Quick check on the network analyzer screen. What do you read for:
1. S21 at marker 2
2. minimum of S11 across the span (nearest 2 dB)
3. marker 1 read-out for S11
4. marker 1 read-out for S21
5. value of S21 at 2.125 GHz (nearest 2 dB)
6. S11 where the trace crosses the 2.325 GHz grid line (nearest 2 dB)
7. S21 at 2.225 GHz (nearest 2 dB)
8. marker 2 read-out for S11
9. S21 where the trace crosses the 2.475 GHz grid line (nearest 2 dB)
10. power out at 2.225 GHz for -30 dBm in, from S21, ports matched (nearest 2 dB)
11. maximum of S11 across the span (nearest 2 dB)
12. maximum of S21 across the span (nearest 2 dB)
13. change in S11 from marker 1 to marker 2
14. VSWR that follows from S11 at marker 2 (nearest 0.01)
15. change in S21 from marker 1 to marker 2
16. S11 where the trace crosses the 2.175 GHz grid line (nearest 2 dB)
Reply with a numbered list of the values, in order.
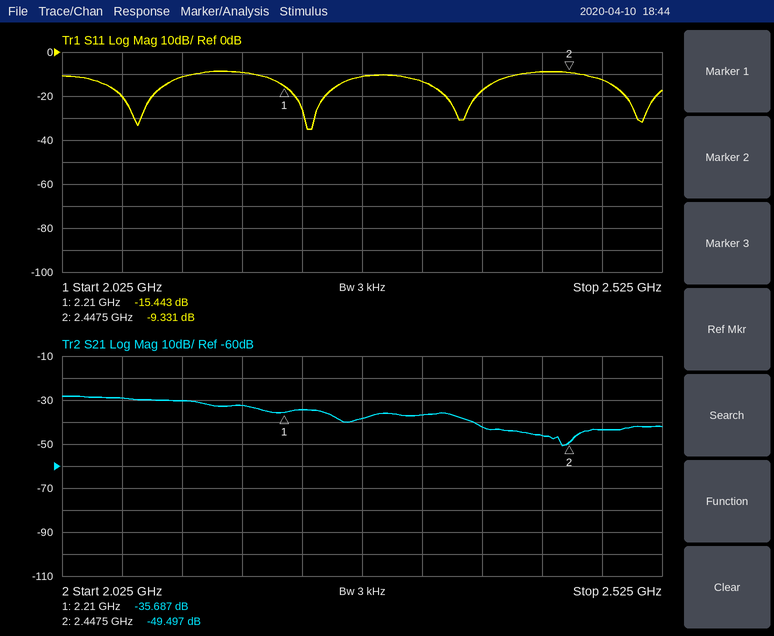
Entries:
1. -49.497 dB
2. -36 dB
3. -15.443 dB
4. -35.687 dB
5. -30 dB
6. -14 dB
7. -34 dB
8. -9.331 dB
9. -44 dB
10. -64 dBm
11. -8 dB
12. -28 dB
13. 6.112 dB
14. 2.04
15. -13.810 dB
16. -10 dB
